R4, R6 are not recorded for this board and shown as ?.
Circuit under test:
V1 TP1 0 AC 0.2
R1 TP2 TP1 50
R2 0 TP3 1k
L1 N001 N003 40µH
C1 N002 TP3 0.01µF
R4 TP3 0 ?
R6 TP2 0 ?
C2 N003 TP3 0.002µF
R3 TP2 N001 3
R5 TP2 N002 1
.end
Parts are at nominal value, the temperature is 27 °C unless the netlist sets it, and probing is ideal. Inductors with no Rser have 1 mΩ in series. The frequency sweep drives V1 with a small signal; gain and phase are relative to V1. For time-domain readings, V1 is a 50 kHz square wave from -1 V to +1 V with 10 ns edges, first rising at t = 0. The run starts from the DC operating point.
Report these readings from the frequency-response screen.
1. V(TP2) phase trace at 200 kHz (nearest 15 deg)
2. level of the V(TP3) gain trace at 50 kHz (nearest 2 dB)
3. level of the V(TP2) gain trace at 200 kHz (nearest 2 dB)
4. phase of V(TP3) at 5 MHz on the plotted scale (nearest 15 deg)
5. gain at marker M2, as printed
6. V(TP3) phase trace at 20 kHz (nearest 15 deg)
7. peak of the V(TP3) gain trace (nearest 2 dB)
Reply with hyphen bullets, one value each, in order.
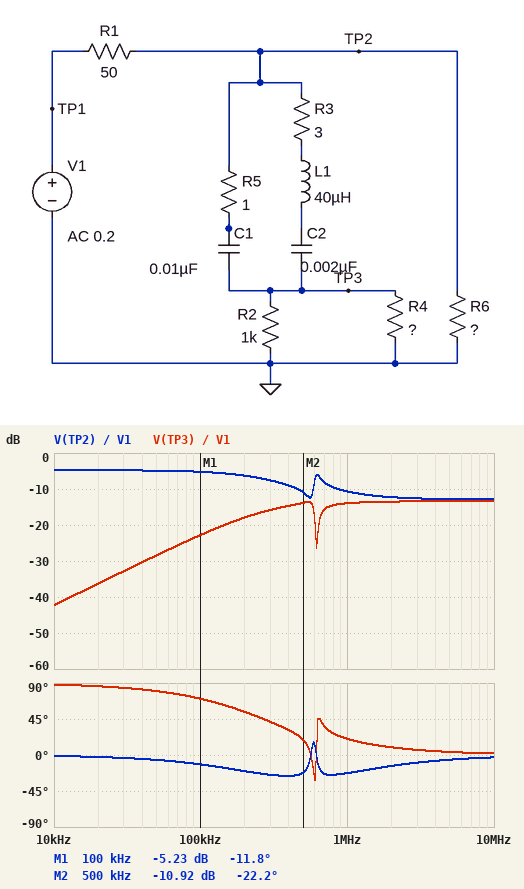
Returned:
- -15 deg
- -28 dB
- -6 dB
- 0 deg
- -10.92 dB
- 90 deg
- -14 dB
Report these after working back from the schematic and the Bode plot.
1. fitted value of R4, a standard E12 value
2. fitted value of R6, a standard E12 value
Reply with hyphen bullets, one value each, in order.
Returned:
- 18 Ω
- 68 Ω
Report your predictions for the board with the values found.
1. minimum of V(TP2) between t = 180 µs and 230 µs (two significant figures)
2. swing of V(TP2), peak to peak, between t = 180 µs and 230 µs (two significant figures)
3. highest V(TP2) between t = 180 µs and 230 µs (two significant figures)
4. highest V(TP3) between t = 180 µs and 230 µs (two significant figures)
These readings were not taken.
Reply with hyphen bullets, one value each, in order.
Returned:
- -600 mV
- 1.2 V
- 600 mV
- 430 mV
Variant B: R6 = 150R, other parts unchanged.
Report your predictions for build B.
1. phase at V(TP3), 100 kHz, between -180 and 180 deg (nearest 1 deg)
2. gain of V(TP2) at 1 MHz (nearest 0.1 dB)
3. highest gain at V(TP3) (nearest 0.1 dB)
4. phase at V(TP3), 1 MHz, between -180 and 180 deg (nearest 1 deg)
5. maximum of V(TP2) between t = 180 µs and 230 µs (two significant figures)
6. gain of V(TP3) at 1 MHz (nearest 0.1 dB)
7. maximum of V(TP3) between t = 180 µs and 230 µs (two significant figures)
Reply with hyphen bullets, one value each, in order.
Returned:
- 67 deg
- -9.7 dB
- -12.5 dB
- 17 deg
- 780 mV
- -13.0 dB
- 470 mV
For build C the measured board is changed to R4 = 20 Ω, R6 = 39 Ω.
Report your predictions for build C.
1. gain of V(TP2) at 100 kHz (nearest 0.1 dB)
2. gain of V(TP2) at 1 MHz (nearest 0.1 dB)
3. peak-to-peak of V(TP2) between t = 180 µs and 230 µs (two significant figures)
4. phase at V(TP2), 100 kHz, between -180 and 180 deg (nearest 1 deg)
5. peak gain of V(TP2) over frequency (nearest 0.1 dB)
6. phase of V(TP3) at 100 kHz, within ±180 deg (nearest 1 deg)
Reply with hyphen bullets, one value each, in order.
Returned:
- -7.5 dB
- -11.8 dB
- 910 mV
- -9 deg
- -7.2 dB
- 72 deg
